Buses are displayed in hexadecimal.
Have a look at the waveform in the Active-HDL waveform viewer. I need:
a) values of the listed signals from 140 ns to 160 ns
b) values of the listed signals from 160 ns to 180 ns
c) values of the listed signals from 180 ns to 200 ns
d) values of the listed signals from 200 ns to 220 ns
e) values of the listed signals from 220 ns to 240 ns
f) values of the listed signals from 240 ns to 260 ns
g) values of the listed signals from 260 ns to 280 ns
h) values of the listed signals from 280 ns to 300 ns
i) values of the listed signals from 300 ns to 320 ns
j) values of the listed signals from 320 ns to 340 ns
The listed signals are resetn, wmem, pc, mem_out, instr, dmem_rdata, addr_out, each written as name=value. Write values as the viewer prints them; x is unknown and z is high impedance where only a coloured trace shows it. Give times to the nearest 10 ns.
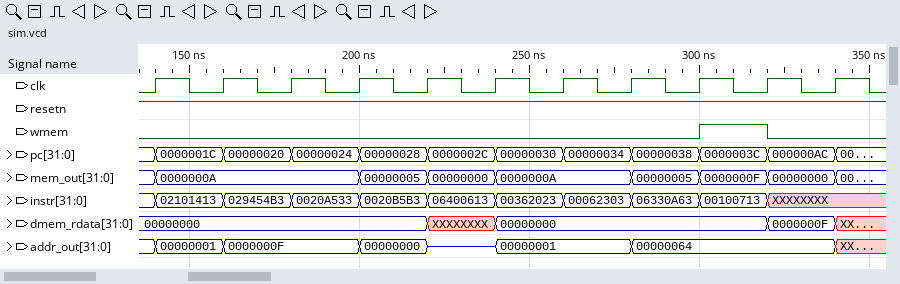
resetn=1, wmem=0, pc=0000001C, mem_out=0000000A, instr=02101413, dmem_rdata=00000000, addr_out=00000001
resetn=1, wmem=0, pc=00000020, mem_out=0000000A, instr=029454B3, dmem_rdata=00000000, addr_out=0000000F
resetn=1, wmem=0, pc=00000024, mem_out=0000000A, instr=0020A533, dmem_rdata=00000000, addr_out=0000000F
resetn=1, wmem=0, pc=00000028, mem_out=00000005, instr=0020B5B3, dmem_rdata=00000000, addr_out=00000000
resetn=1, wmem=0, pc=0000002C, mem_out=00000000, instr=06400613, dmem_rdata=XXXXXXXX, addr_out=z
resetn=1, wmem=0, pc=00000030, mem_out=0000000A, instr=00362023, dmem_rdata=00000000, addr_out=00000001
resetn=1, wmem=0, pc=00000034, mem_out=0000000A, instr=00062303, dmem_rdata=00000000, addr_out=00000001
resetn=1, wmem=0, pc=00000038, mem_out=00000005, instr=06330A63, dmem_rdata=00000000, addr_out=00000064
resetn=1, wmem=1, pc=0000003C, mem_out=0000000F, instr=00100713, dmem_rdata=00000000, addr_out=00000064
resetn=1, wmem=0, pc=000000AC, mem_out=00000000, instr=XXXXXXXX, dmem_rdata=0000000F, addr_out=00000064
